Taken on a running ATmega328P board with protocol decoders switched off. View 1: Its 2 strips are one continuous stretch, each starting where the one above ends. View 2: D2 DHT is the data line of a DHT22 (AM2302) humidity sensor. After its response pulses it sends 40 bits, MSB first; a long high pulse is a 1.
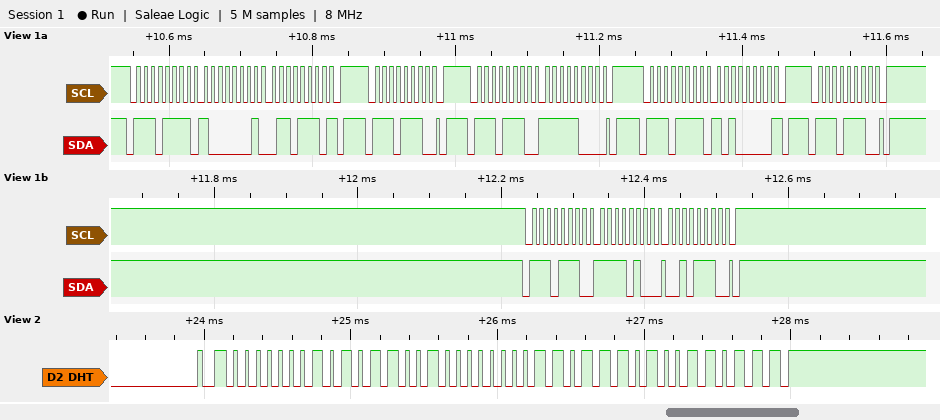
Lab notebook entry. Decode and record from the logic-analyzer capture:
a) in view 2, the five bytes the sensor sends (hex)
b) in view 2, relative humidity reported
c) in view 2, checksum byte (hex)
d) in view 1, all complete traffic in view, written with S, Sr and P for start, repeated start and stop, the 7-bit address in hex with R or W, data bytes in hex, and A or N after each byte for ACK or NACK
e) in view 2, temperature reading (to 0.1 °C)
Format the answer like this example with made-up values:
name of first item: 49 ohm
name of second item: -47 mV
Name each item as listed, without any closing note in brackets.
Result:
in view 2, the five bytes the sensor sends: 01 59 00 DD 37
in view 2, relative humidity reported: 34.5 %
in view 2, checksum byte: 0x37
in view 1, all complete traffic in view, written with S, Sr and P for start, repeated start and stop, the 7-bit address in hex with R or W, data bytes in hex, and A or N after each byte for ACK or NACK: S 77R A 81 A 6E N P S 77W A P S 77W A F8 A P S 77R A A0 N P S 77W A P S 77W A F4 A 2E A P
in view 2, temperature reading: 22.1 °C
